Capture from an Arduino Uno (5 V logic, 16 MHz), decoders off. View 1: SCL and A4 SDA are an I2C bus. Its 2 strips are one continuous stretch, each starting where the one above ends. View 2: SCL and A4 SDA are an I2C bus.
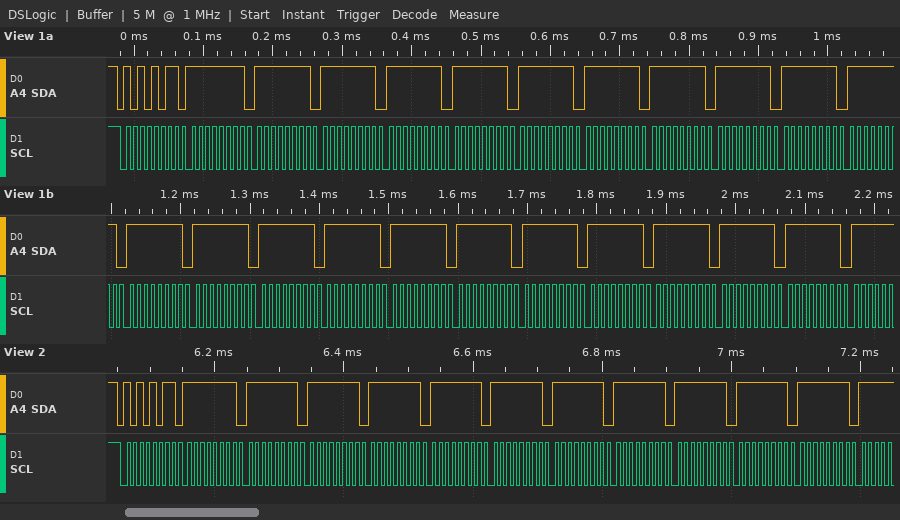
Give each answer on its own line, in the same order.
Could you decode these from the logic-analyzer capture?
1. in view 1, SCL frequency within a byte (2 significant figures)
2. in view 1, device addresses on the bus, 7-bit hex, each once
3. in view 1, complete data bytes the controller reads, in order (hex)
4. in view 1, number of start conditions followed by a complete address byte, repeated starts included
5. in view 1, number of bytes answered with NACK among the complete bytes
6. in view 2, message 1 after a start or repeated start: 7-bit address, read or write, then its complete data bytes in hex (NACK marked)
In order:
100 kHz
0x55
FF FF FF FF FF FF FF FF FF FF FF FF FF FF FF FF FF FF FF FF FF FF
1
0
0x55 read: FF FF FF FF FF FF FF FF FF FF FF
